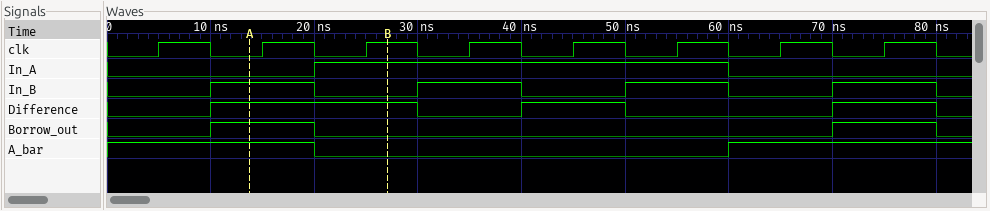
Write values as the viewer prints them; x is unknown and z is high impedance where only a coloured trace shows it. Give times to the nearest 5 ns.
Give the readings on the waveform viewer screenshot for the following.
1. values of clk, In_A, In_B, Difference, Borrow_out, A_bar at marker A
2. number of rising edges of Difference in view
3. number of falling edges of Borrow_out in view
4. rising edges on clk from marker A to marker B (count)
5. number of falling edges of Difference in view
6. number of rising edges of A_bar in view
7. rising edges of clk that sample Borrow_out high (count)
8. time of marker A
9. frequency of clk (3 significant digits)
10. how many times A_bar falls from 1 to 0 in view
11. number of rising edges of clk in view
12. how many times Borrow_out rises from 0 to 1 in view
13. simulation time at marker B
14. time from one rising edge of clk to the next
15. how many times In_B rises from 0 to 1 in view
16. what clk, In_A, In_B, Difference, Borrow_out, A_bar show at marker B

clk=0, In_A=0, In_B=1, Difference=1, Borrow_out=1, A_bar=1
3
2
2
3
1
2
15 ns
100 MHz
1
8
2
25 ns
10 ns
4
clk=1, In_A=1, In_B=0, Difference=1, Borrow_out=0, A_bar=0
